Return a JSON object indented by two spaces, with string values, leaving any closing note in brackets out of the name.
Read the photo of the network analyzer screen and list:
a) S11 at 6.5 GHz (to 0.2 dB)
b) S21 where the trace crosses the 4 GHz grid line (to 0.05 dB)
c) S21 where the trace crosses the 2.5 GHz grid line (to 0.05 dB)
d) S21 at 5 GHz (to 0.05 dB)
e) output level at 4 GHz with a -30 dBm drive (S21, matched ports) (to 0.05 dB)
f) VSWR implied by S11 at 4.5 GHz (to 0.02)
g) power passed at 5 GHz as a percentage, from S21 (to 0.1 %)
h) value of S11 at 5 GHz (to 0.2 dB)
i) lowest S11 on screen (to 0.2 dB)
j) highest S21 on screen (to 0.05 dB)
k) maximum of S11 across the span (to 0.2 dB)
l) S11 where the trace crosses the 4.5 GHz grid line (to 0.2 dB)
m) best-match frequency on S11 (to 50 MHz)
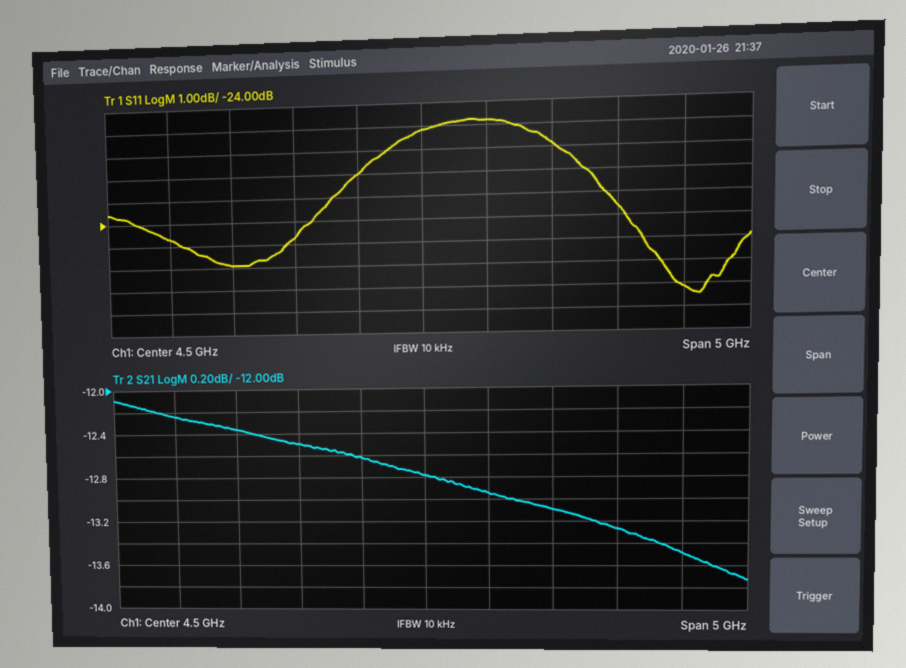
{
  "S11 at 6.5 GHz": "-27.2 dB",
  "S21 where the trace crosses the 4 GHz grid line": "-12.60 dB",
  "S21 where the trace crosses the 2.5 GHz grid line": "-12.25 dB",
  "S21 at 5 GHz": "-12.95 dB",
  "output level at 4 GHz with a -30 dBm drive (S21, matched ports)": "-42.60 dBm",
  "VSWR implied by S11 at 4.5 GHz": "1.22",
  "power passed at 5 GHz as a percentage, from S21": "5.1 %",
  "value of S11 at 5 GHz": "-19.8 dB",
  "lowest S11 on screen": "-27.4 dB",
  "highest S21 on screen": "-12.10 dB",
  "maximum of S11 across the span": "-19.8 dB",
  "S11 where the trace crosses the 4.5 GHz grid line": "-20.2 dB",
  "best-match frequency on S11": "6.60 GHz"
}
